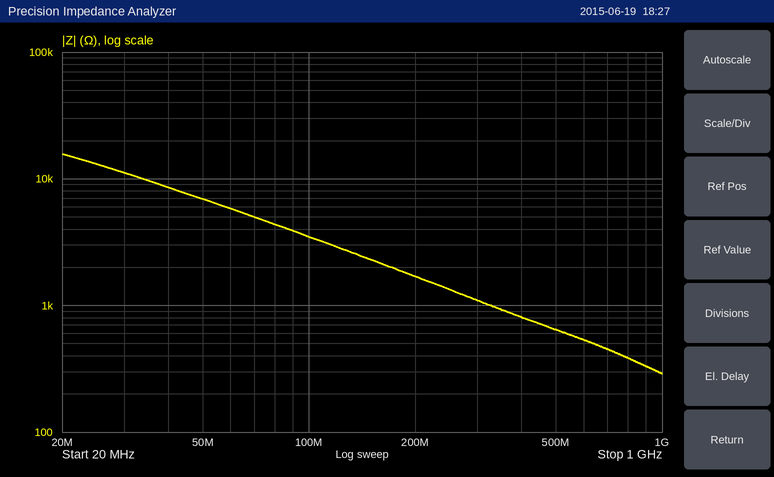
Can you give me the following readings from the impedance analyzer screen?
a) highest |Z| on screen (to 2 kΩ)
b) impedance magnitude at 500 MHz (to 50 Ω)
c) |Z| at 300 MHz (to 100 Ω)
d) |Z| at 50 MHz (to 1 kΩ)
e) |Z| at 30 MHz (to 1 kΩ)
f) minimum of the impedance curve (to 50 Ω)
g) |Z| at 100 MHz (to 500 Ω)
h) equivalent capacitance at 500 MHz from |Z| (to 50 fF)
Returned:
16 kΩ
650 Ω
1.1 kΩ
7 kΩ
11 kΩ
300 Ω
3.5 kΩ
500 fF
